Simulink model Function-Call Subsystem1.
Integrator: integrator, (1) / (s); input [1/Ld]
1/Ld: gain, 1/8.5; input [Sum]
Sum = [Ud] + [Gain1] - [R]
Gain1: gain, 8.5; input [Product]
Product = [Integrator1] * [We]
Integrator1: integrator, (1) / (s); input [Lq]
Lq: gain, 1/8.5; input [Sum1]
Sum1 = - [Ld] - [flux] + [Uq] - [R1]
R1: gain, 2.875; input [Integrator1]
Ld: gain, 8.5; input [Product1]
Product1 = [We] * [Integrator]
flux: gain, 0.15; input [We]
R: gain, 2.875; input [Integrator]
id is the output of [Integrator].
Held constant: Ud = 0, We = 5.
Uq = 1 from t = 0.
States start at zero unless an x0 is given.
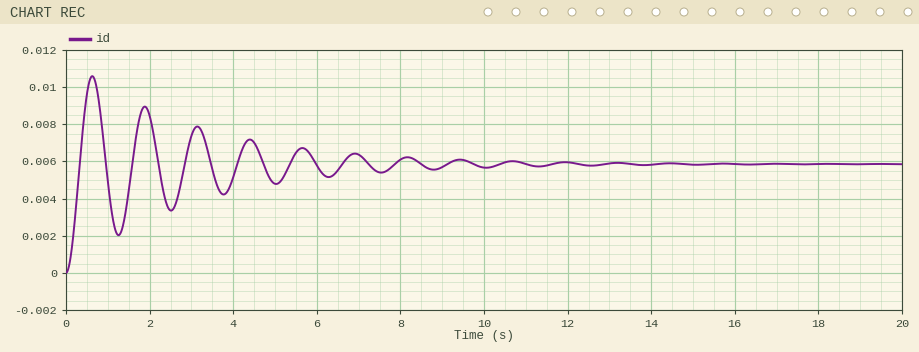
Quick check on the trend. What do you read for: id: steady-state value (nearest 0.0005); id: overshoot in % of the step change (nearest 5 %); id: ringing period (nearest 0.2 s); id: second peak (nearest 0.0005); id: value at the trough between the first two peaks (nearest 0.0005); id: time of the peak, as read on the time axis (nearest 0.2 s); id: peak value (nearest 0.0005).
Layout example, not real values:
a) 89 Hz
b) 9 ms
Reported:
a) 0.0060
b) 80 %
c) 1.2 s
d) 0.0090
e) 0.0020
f) 0.6 s
g) 0.0105
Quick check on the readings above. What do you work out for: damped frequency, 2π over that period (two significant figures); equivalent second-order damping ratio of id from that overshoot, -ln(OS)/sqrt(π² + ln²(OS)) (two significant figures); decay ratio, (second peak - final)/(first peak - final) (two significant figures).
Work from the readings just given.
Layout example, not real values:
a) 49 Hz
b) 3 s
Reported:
a) 5.2 rad/s
b) 0.071
c) 0.67
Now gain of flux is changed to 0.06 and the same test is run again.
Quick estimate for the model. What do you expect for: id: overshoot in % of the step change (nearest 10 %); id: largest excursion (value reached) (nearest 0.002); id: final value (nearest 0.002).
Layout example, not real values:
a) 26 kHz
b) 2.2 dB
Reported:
a) 80 %
b) 0.030
c) 0.016
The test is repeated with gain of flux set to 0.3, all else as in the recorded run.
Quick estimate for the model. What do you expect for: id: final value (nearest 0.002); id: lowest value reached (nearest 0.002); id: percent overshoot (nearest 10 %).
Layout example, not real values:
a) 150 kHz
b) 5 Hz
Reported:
a) -0.012
b) -0.022
c) 80 %
